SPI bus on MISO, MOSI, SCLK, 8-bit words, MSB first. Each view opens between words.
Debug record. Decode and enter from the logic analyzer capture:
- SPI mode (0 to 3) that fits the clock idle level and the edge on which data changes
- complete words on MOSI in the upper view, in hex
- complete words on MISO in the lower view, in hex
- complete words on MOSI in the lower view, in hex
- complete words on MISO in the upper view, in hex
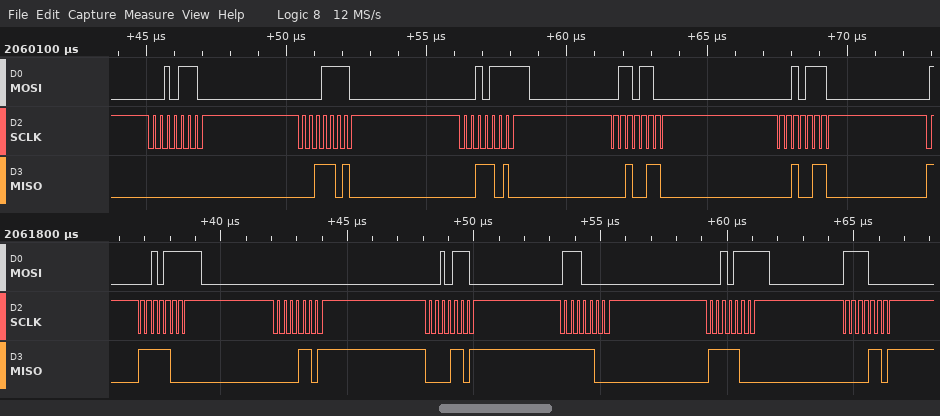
3
2E, 1E, 2F, 6C, 2E
F8, 0D, 0D, F8, F8, 0D
2F, 00, 2E, E0, 2F, F0
00, 3A, 3A, 26, 26
